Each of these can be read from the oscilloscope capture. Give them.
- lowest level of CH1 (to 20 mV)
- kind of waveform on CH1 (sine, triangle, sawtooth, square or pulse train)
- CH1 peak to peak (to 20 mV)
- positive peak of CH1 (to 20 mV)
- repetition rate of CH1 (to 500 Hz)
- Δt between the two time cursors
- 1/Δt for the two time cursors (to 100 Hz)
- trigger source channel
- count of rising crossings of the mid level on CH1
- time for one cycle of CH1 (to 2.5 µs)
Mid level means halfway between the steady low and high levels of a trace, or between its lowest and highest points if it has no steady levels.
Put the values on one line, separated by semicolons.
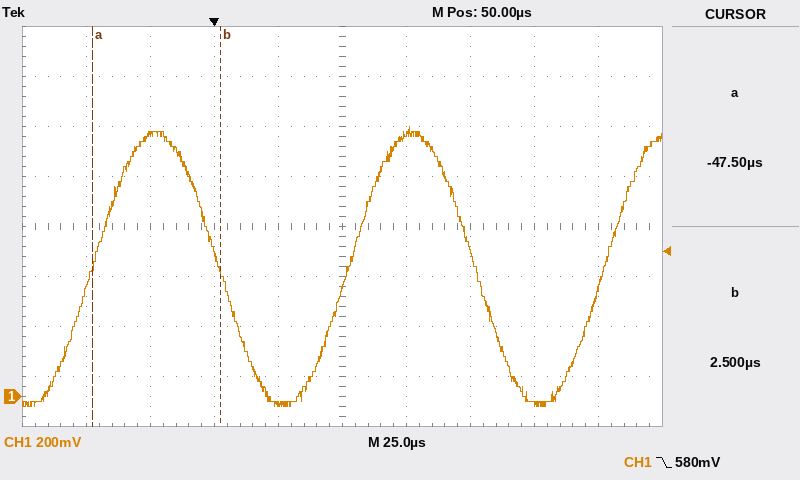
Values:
-40 mV; sine; 1.12 V; 1.08 V; 10.0 kHz; 50.0 µs; 20.0 kHz; CH1; 3; 100.0 µs
